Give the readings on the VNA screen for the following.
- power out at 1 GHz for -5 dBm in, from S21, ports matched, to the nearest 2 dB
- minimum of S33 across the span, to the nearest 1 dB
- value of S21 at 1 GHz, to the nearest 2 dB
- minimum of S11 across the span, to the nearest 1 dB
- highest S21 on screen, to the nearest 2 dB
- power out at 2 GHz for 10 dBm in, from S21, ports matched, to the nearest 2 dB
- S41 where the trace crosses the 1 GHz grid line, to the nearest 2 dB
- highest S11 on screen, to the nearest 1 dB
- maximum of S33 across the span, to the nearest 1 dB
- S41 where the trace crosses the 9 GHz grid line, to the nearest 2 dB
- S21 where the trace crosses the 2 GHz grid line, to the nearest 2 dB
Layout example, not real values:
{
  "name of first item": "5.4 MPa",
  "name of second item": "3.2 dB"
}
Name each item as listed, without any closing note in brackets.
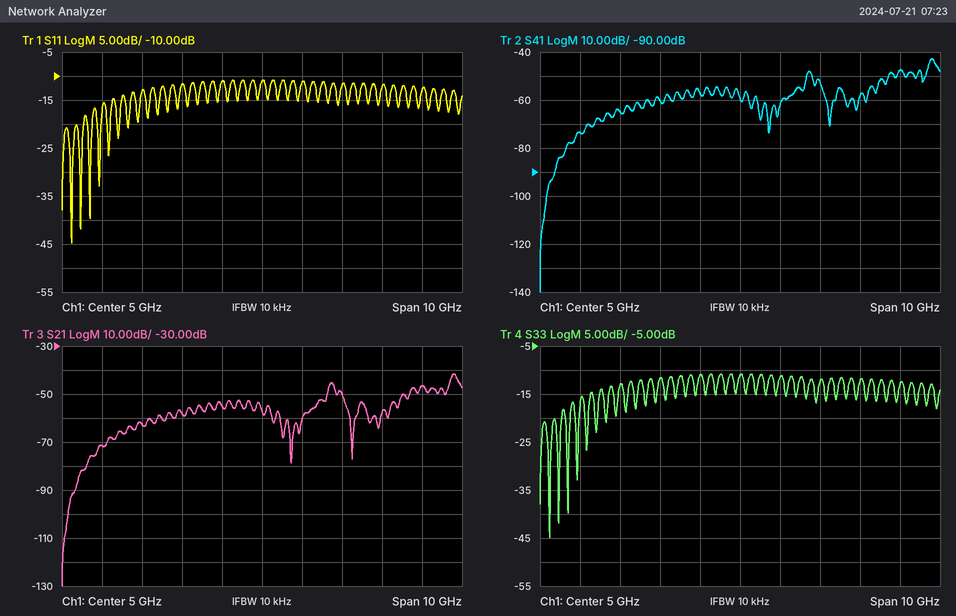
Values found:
{
  "power out at 1 GHz for -5 dBm in, from S21, ports matched, to the nearest 2 dB": "-76 dBm",
  "minimum of S33 across the span, to the nearest 1 dB": "-45 dB",
  "value of S21 at 1 GHz, to the nearest 2 dB": "-72 dB",
  "minimum of S11 across the span, to the nearest 1 dB": "-45 dB",
  "highest S21 on screen, to the nearest 2 dB": "-42 dB",
  "power out at 2 GHz for 10 dBm in, from S21, ports matched, to the nearest 2 dB": "-52 dBm",
  "S41 where the trace crosses the 1 GHz grid line, to the nearest 2 dB": "-74 dB",
  "highest S11 on screen, to the nearest 1 dB": "-11 dB",
  "maximum of S33 across the span, to the nearest 1 dB": "-11 dB",
  "S41 where the trace crosses the 9 GHz grid line, to the nearest 2 dB": "-48 dB",
  "S21 where the trace crosses the 2 GHz grid line, to the nearest 2 dB": "-62 dB"
}
